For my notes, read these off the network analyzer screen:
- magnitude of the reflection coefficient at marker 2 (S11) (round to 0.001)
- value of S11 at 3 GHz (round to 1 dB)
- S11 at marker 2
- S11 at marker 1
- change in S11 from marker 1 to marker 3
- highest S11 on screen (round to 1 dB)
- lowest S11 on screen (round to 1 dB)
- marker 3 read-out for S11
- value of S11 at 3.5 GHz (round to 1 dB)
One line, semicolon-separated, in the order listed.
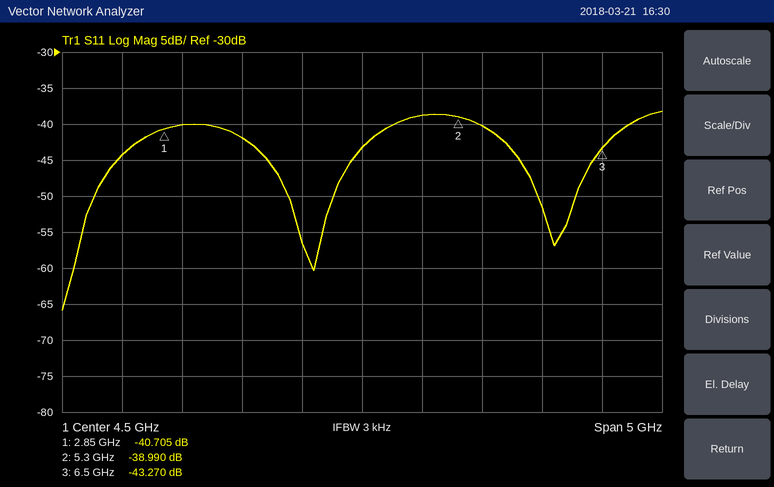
0.011; -40 dB; -38.990 dB; -40.705 dB; -2.565 dB; -38 dB; -66 dB; -43.270 dB; -42 dB
